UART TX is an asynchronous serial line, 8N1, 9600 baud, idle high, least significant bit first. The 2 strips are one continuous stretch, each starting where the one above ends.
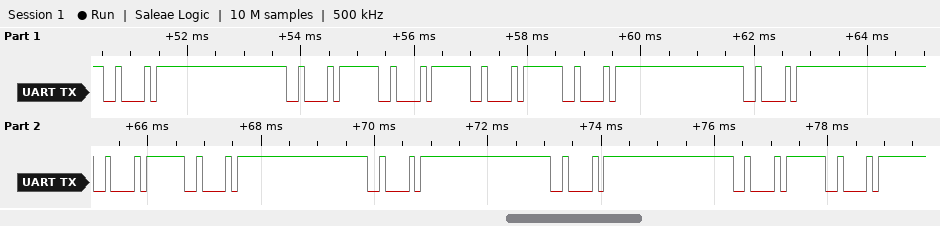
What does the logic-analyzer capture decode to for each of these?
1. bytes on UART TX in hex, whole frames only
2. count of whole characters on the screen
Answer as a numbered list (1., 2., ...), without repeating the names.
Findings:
1. 0x42 0x42 0x42 0x42 0x42 0x42 0x42 0x42 0x42 0x42 0x42 0x42
2. 12
